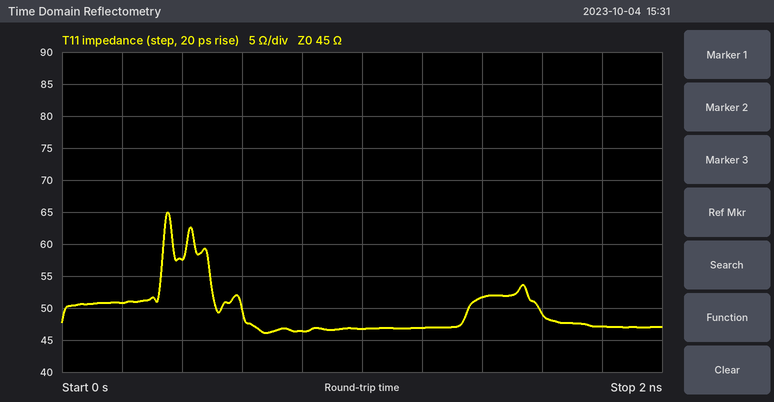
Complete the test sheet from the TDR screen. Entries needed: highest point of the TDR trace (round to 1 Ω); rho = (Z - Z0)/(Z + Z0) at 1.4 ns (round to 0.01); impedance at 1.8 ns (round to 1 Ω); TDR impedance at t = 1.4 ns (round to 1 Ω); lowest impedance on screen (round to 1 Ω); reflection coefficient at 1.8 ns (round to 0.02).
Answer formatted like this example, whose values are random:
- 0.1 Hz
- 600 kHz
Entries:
- 65 Ω
- +0.07
- 47 Ω
- 52 Ω
- 46 Ω
- +0.02
